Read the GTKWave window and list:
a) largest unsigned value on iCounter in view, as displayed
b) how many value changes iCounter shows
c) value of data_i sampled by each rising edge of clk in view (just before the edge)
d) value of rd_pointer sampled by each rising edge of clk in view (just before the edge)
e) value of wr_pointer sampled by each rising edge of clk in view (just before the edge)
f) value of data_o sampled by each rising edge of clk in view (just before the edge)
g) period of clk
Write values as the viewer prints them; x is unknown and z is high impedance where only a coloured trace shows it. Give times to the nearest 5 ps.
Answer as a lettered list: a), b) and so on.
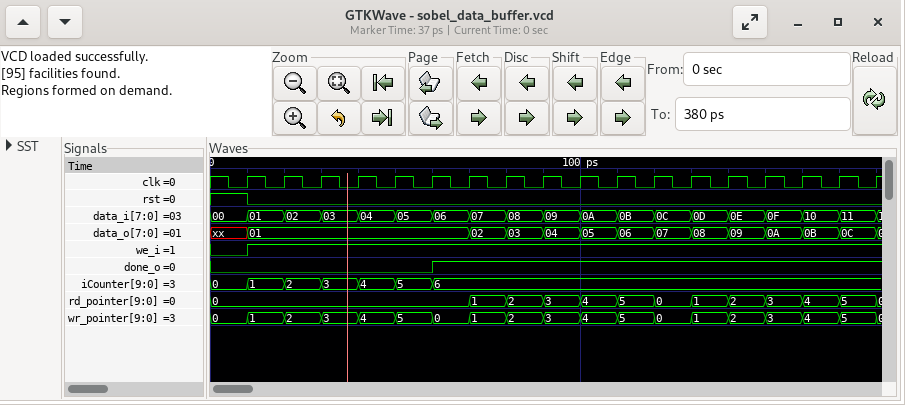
a) 6
b) 6
c) 00, 01, 02, 03, 04, 05, 06, 07, 08, 09, 0A, 0B, 0C, 0D, 0E, 0F, 10, 11
d) 0, 0, 0, 0, 0, 0, 0, 1, 2, 3, 4, 5, 0, 1, 2, 3, 4, 5
e) 0, 1, 2, 3, 4, 5, 0, 1, 2, 3, 4, 5, 0, 1, 2, 3, 4, 5
f) xx, 01, 01, 01, 01, 01, 01, 02, 03, 04, 05, 06, 07, 08, 09, 0A, 0B, 0C
g) 10 ps
